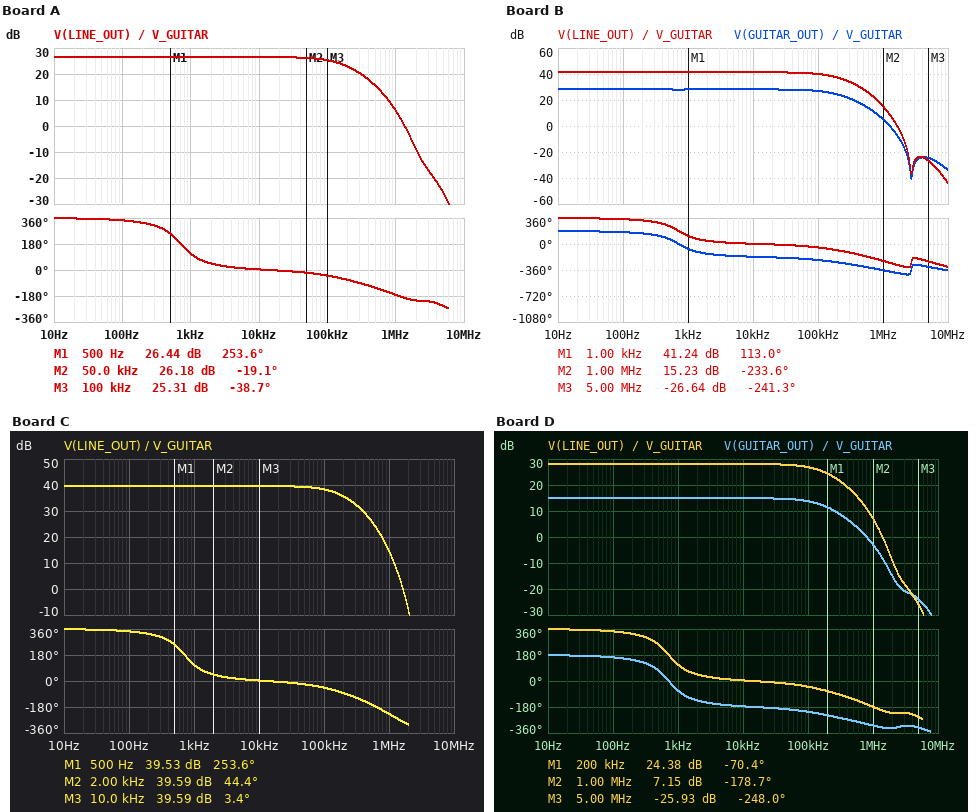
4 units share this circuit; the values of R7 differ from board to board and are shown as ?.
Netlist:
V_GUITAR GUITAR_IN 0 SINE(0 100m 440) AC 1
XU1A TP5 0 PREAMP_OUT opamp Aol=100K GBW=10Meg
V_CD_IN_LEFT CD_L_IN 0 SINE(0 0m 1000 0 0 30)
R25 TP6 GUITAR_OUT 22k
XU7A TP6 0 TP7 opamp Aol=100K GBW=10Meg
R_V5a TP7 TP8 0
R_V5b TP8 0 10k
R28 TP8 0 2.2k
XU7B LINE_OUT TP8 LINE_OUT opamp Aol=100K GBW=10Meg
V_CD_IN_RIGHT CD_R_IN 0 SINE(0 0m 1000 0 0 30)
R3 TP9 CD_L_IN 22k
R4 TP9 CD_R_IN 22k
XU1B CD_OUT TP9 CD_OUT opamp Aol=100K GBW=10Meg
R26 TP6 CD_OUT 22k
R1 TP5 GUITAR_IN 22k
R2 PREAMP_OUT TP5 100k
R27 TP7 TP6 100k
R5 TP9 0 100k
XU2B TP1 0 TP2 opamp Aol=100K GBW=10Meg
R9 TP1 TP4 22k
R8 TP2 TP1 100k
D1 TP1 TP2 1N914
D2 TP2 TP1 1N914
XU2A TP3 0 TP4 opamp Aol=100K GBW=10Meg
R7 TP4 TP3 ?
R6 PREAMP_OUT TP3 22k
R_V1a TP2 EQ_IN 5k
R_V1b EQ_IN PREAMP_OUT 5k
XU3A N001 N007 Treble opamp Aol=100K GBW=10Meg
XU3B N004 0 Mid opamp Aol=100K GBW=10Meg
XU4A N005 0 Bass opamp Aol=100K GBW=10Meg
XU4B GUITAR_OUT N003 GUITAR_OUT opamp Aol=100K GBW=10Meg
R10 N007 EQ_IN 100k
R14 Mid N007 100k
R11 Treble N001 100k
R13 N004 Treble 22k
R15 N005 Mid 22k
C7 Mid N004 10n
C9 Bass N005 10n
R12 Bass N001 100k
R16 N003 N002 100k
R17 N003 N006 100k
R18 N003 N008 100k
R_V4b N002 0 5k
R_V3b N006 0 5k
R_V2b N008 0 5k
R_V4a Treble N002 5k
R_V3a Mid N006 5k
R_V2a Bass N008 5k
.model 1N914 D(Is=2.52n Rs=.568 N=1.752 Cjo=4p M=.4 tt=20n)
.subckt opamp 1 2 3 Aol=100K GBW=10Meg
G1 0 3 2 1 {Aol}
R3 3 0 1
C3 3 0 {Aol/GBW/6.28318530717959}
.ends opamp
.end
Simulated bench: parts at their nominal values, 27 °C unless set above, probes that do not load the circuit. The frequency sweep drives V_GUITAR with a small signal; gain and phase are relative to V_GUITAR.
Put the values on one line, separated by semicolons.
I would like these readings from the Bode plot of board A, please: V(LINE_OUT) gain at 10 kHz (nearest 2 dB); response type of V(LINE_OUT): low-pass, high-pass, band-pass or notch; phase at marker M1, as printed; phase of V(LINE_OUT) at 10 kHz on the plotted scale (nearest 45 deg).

26 dB; low-pass; 253.6 deg; 0 deg
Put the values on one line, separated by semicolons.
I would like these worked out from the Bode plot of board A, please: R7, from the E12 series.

56 kΩ
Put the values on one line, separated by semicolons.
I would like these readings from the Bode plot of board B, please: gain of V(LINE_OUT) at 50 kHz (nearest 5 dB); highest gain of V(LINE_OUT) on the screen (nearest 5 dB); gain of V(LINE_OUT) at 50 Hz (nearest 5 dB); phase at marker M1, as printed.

40 dB; 40 dB; 40 dB; 113.0 deg
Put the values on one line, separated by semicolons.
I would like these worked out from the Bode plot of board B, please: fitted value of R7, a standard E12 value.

330 kΩ
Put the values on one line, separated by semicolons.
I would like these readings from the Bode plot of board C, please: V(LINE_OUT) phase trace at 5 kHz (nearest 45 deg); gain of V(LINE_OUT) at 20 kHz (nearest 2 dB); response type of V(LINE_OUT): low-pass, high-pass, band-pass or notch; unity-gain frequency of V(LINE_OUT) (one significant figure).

0 deg; 40 dB; low-pass; 2 MHz
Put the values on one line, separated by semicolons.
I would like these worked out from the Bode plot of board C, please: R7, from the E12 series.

270 kΩ
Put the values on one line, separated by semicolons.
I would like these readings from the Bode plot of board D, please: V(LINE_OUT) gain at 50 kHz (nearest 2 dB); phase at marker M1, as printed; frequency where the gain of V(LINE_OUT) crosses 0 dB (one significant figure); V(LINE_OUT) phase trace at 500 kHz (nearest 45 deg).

28 dB; -70.4 deg; 1 MHz; -135 deg
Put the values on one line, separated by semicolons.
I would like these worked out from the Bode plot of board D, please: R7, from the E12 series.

68 kΩ
